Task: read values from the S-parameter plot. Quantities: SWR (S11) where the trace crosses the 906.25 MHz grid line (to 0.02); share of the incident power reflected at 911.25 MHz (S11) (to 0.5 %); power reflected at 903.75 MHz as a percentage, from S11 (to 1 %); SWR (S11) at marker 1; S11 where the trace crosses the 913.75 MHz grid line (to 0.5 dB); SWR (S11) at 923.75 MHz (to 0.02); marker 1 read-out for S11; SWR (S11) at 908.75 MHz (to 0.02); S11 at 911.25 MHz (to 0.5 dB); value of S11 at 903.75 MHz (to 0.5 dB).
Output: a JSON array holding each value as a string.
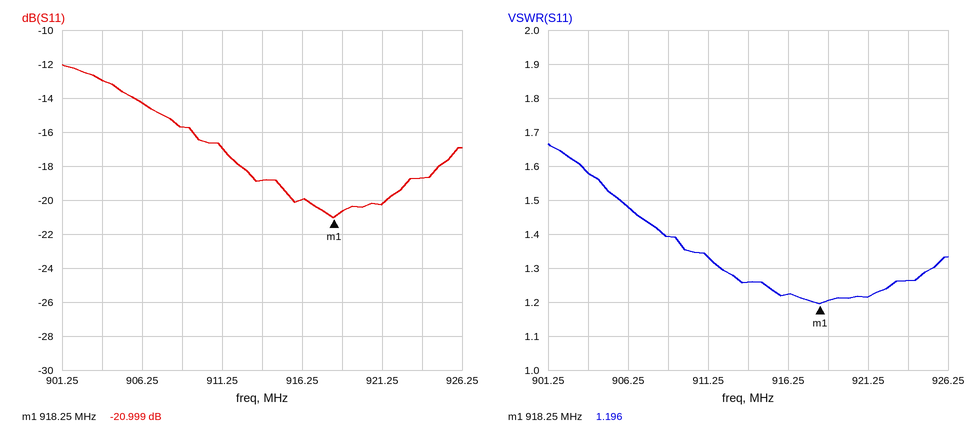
["1.48", "2.0 %", "5 %", "1.196", "-19.0 dB", "1.26", "-20.999 dB", "1.40", "-17.0 dB", "-13.0 dB"]
